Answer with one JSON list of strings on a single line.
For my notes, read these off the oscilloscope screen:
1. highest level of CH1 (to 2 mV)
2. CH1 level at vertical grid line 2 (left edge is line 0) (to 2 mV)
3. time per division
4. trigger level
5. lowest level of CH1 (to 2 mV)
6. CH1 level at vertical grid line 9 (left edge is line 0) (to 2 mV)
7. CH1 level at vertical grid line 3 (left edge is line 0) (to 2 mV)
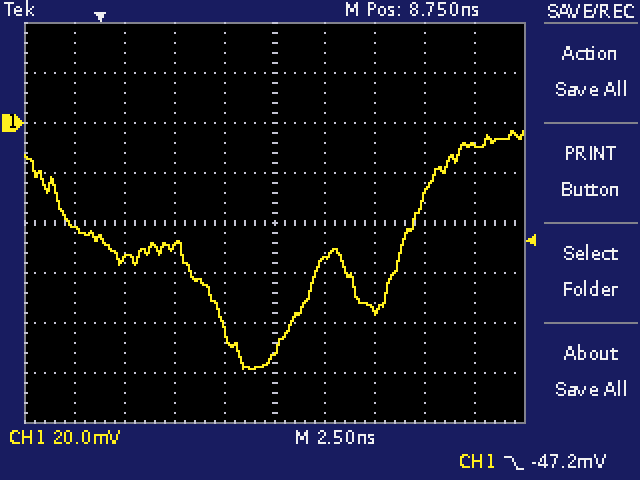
["-4 mV", "-54 mV", "2.5 ns", "-47.2 mV", "-98 mV", "-8 mV", "-50 mV"]
